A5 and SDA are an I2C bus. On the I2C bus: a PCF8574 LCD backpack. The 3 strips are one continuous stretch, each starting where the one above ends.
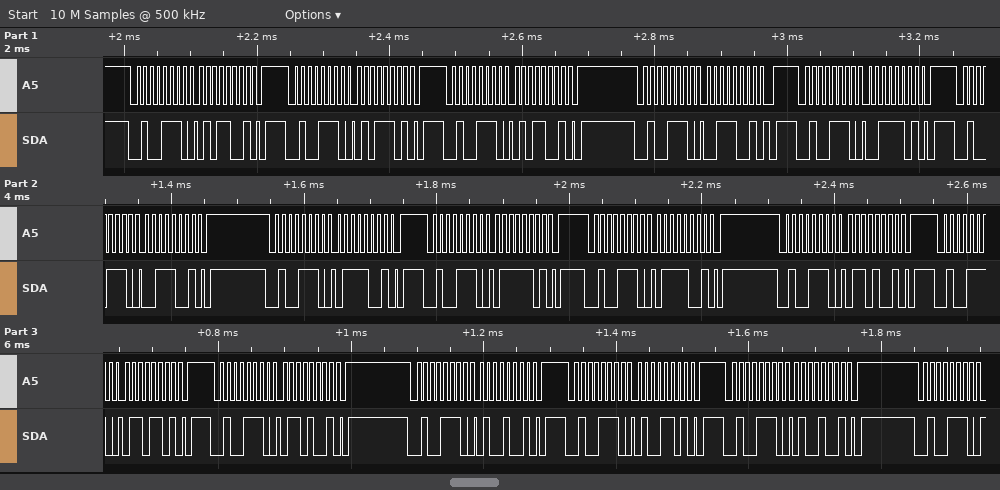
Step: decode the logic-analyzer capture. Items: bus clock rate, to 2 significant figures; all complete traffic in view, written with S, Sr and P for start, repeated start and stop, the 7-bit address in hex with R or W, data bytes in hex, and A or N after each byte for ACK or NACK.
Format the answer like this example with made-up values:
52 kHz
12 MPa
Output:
100 kHz
S 27W A 59 A P S 27W A 5D A P S 27W A 59 A P S 27W A 39 A P S 27W A 3D A P S 27W A 39 A P S 27W A 79 A P S 27W A 7D A P S 27W A 79 A P S 27W A 69 A P S 27W A 6D A P S 27W A 69 A P S 27W A 49 A P S 27W A 4D A P S 27W A 49 A P S 27W A
